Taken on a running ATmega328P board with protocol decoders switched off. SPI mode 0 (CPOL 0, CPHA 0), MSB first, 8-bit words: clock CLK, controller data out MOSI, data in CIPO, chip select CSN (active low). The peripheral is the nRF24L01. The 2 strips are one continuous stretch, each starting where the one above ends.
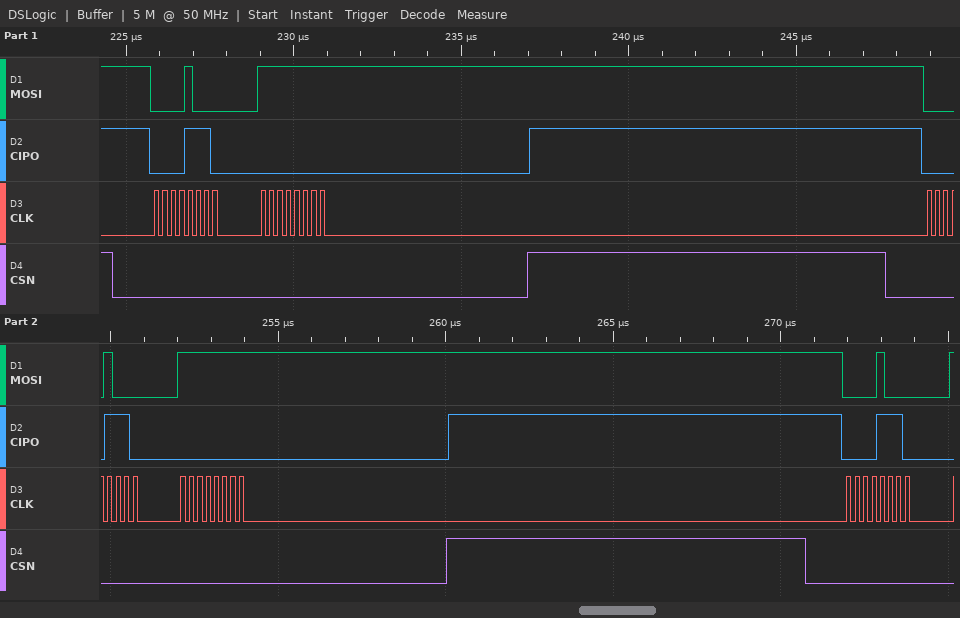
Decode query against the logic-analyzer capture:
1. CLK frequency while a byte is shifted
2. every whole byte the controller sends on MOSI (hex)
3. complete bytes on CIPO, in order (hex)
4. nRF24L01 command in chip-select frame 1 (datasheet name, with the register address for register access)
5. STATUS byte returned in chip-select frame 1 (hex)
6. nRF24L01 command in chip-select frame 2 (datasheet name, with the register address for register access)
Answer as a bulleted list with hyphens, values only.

- 4 MHz
- 08 FF 08 FF 08
- 0E 00 0E 00 0E
- R_REGISTER 0x08
- 0x0E
- R_REGISTER 0x08
